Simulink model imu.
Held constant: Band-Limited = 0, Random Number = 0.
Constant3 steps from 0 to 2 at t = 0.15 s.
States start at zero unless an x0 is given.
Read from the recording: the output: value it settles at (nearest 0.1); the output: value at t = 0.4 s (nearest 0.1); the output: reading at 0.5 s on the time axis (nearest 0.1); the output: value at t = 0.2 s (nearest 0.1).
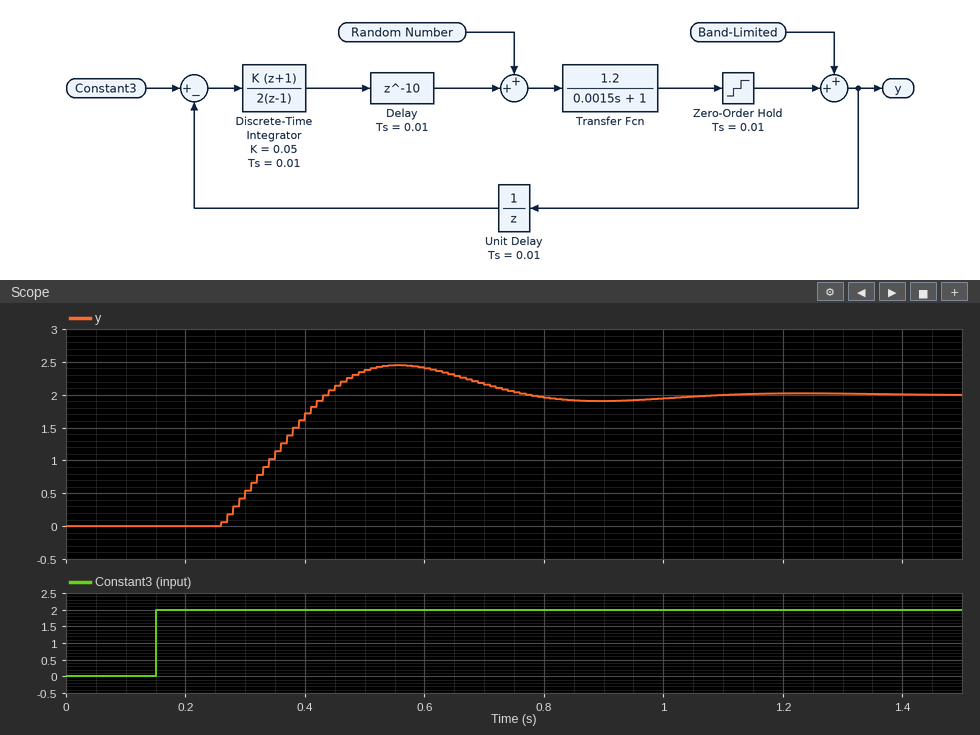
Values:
2.0
1.7
2.4
0.0
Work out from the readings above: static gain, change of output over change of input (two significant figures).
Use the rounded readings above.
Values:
1.0
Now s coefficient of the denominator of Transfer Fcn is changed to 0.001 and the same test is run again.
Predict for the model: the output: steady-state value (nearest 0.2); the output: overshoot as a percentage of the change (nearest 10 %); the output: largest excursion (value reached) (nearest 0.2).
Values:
2.0
20 %
2.4
